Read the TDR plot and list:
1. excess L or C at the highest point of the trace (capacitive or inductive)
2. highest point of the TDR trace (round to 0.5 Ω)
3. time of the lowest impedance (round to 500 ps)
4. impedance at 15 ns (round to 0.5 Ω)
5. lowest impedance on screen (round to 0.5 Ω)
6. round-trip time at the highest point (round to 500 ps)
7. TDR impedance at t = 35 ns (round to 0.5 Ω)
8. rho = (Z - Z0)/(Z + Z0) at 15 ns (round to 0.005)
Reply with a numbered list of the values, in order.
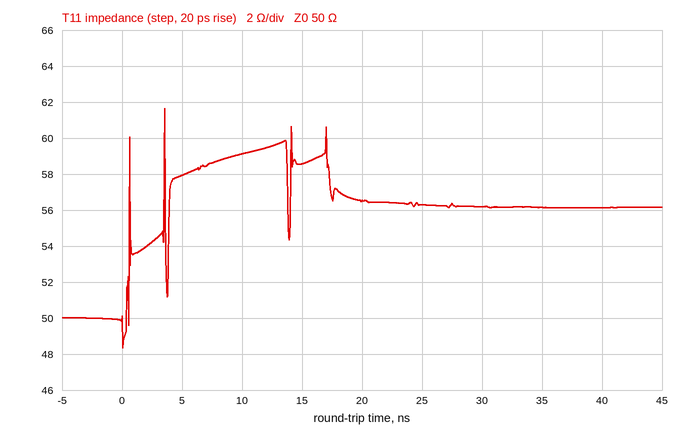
1. inductive
2. 61.5 Ω
3. 0.0 ns
4. 58.5 Ω
5. 48.5 Ω
6. 3.5 ns
7. 56.0 Ω
8. +0.080
